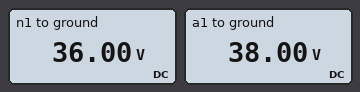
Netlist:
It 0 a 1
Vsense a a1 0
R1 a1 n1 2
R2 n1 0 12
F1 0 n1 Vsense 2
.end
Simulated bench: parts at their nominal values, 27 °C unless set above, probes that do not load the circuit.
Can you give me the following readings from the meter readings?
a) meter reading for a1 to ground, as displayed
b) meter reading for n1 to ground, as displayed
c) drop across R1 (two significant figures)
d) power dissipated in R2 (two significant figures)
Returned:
38.00 V
36.00 V
2.0 V
110 W
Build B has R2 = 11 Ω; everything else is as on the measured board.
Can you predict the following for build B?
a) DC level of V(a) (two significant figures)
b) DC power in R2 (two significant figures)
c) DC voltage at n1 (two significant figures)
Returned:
35 V
99 W
33 V
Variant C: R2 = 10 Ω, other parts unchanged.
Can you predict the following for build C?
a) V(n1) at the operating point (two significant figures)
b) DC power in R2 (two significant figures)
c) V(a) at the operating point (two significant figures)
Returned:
30 V
90 W
32 V
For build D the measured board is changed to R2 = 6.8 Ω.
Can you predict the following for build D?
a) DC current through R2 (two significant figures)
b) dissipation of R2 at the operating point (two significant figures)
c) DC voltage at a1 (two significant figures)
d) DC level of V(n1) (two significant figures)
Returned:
3.0 A
61 W
22 V
20 V
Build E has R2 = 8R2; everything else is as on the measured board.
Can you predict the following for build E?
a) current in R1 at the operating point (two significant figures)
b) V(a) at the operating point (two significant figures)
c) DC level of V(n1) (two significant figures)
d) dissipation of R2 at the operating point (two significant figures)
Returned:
1.0 A
27 V
25 V
74 W
